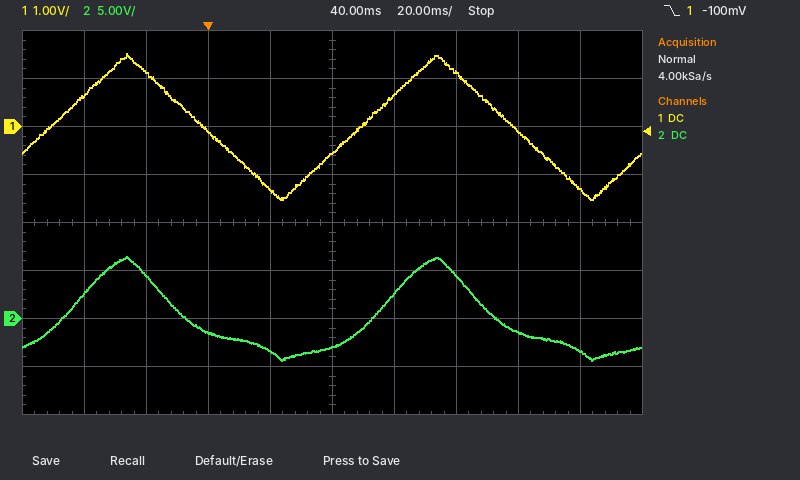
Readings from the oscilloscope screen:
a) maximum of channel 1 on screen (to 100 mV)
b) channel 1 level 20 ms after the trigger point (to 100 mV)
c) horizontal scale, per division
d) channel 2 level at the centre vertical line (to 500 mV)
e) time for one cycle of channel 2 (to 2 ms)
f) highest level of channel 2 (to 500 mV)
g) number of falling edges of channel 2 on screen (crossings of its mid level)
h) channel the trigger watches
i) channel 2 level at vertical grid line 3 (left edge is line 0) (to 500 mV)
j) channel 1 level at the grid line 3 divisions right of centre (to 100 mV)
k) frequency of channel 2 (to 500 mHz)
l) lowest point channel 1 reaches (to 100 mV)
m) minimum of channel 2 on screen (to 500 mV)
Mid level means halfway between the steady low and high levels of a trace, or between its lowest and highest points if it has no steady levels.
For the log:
1.5 V
-1.3 V
20 ms
-3.0 V
100 ms
6.5 V
2
channel 1
-1.5 V
-100 mV
10.0 Hz
-1.5 V
-4.5 V
